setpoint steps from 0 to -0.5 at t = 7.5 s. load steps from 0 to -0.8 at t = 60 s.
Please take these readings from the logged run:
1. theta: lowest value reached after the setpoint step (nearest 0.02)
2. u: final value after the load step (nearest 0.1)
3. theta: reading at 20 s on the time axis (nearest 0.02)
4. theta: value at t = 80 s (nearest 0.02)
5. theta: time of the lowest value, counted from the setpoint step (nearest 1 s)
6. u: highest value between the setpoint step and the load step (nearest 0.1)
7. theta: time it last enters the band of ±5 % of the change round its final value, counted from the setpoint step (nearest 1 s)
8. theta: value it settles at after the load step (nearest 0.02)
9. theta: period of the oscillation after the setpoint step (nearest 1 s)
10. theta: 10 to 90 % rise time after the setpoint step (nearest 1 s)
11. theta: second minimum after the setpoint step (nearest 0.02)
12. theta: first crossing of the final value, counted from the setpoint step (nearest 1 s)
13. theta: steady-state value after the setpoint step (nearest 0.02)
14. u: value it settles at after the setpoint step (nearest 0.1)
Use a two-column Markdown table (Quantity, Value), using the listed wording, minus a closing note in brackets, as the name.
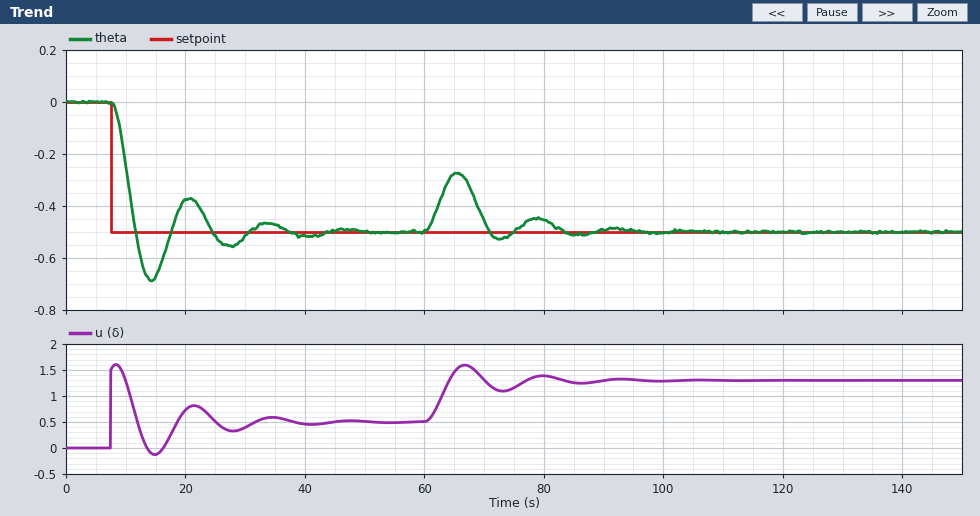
| Quantity | Value |
|---|---|
| theta: lowest value reached after the setpoint step | -0.68 |
| u: final value after the load step | 1.3 |
| theta: reading at 20 s on the time axis | -0.38 |
| theta: value at t = 80 s | -0.46 |
| theta: time of the lowest value, counted from the setpoint step | 7 s |
| u: highest value between the setpoint step and the load step | 1.6 |
| theta: time it last enters the band of ±5 % of the change round its final value, counted from the setpoint step | 28 s |
| theta: value it settles at after the load step | -0.50 |
| theta: period of the oscillation after the setpoint step | 13 s |
| theta: 10 to 90 % rise time after the setpoint step | 3 s |
| theta: second minimum after the setpoint step | -0.56 |
| theta: first crossing of the final value, counted from the setpoint step | 4 s |
| theta: steady-state value after the setpoint step | -0.50 |
| u: value it settles at after the setpoint step | 0.5 |
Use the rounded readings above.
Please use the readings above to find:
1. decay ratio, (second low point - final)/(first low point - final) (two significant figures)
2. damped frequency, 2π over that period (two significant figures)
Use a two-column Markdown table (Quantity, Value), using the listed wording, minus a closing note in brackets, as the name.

| Quantity | Value |
|---|---|
| decay ratio, (second low point - final)/(first low point - final) | 0.33 |
| damped frequency, 2π over that period | 0.48 rad/s |
